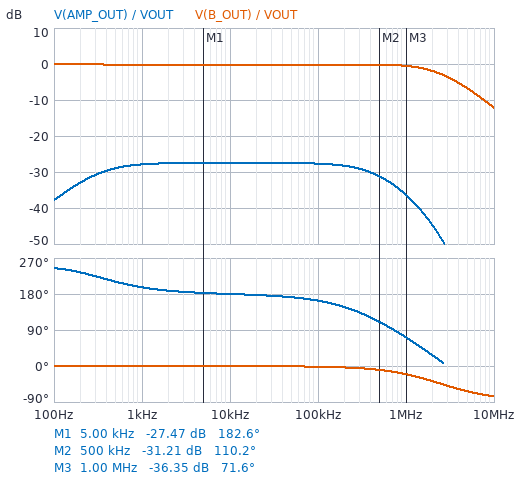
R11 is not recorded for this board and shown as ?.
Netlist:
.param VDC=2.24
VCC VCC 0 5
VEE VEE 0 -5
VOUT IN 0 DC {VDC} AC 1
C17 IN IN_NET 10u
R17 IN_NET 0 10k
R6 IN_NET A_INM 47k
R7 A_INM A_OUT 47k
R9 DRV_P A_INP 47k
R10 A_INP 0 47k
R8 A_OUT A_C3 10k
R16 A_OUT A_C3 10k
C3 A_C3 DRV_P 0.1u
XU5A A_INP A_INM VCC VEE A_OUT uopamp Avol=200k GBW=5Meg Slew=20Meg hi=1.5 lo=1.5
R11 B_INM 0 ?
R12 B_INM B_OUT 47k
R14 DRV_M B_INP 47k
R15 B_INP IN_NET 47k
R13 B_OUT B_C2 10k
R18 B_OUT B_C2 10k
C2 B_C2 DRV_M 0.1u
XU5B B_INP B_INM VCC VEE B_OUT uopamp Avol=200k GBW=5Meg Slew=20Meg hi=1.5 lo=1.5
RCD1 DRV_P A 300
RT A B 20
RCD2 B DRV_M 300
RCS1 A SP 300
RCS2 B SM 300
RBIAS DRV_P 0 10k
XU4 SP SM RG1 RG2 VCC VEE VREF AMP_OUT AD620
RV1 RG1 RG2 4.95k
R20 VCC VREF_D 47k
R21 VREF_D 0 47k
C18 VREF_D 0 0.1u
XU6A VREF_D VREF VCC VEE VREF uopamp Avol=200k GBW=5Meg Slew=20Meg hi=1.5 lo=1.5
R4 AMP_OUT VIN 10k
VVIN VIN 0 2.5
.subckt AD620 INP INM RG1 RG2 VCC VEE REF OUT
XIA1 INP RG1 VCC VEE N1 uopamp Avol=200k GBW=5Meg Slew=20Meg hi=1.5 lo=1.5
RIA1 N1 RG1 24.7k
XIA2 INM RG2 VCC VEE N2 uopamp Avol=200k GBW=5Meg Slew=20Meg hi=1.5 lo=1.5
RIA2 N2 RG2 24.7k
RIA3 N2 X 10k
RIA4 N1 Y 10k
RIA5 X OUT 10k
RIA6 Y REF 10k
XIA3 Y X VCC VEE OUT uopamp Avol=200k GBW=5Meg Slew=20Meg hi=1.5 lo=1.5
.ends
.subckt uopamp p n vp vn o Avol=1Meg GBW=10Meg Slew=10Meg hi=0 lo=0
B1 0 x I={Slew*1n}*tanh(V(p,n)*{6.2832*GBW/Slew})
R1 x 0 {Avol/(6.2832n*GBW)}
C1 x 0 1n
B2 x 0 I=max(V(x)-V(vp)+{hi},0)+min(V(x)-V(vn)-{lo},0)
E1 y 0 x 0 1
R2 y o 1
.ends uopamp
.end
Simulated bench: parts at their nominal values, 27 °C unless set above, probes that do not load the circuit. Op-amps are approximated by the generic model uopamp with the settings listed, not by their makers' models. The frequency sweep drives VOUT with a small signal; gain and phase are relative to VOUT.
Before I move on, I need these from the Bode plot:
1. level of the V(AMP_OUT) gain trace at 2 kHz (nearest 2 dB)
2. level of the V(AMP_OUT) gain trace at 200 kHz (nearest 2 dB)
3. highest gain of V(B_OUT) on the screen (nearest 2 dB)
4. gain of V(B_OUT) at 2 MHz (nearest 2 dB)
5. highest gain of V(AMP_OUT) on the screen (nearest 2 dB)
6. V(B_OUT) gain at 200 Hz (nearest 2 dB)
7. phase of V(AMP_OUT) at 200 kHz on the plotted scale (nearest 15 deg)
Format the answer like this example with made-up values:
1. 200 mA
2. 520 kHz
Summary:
1. -28 dB
2. -28 dB
3. 0 dB
4. -2 dB
5. -28 dB
6. 0 dB
7. 150 deg
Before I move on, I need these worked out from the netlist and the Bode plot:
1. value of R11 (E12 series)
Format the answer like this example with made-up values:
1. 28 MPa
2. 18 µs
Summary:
1. 56 kΩ
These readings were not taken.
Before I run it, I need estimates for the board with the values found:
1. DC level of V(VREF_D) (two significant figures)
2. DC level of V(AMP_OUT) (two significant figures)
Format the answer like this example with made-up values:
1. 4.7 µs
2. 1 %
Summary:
1. 2.5 V
2. 2.5 V
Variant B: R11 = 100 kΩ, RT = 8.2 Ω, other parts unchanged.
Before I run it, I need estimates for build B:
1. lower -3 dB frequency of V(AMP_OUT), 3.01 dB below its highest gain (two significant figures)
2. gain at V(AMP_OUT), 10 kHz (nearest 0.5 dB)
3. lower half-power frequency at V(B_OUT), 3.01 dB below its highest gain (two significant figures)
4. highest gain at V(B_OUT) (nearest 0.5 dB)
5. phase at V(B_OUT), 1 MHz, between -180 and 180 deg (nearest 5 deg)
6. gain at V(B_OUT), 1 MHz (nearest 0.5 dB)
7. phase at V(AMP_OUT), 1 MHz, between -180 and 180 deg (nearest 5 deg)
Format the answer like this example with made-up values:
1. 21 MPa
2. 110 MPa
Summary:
1. 330 Hz
2. -36.5 dB
3. 2.0 Hz
4. -2.0 dB
5. -10 deg
6. -3.0 dB
7. 75 deg
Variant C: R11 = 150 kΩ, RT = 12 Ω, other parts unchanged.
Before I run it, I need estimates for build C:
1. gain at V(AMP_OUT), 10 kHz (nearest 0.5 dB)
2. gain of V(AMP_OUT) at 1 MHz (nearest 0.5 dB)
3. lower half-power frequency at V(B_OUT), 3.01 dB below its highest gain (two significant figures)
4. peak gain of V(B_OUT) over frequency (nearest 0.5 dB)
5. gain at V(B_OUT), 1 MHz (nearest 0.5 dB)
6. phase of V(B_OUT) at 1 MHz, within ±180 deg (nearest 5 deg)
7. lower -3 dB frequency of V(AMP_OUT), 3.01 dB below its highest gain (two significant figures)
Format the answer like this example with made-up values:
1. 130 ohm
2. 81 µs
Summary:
1. -33.5 dB
2. -42.5 dB
3. 2.0 Hz
4. -3.0 dB
5. -4.0 dB
6. -5 deg
7. 340 Hz
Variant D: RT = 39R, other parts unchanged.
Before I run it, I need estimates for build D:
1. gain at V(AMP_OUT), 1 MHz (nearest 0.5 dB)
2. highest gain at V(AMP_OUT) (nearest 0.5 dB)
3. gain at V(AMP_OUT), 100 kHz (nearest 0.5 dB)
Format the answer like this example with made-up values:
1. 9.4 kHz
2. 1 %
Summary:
1. -30.5 dB
2. -21.5 dB
3. -22.0 dB
